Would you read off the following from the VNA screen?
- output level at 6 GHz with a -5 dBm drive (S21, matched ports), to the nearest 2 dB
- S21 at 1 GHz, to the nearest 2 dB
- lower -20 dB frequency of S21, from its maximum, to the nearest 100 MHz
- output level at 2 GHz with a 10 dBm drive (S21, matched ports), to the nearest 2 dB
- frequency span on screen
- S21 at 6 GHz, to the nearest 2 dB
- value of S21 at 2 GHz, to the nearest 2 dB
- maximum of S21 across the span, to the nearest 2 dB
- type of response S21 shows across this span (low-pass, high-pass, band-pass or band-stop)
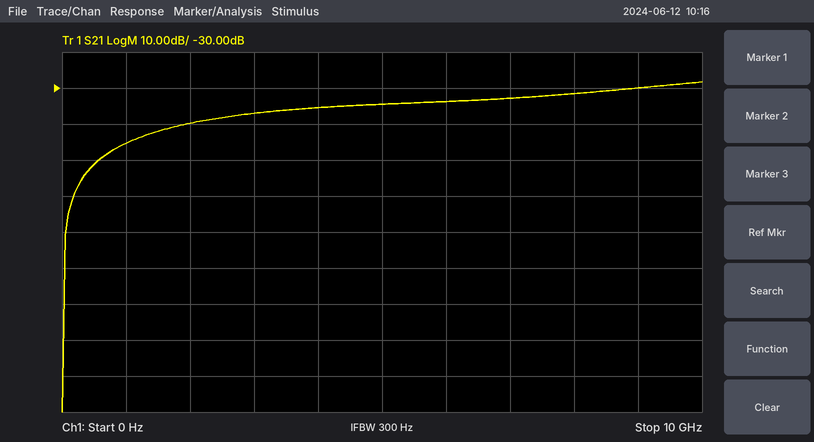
-38 dBm
-46 dB
700 MHz
-30 dBm
10 GHz
-34 dB
-40 dB
-28 dB
high-pass
